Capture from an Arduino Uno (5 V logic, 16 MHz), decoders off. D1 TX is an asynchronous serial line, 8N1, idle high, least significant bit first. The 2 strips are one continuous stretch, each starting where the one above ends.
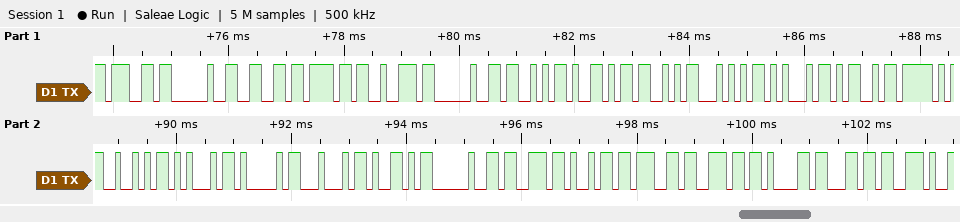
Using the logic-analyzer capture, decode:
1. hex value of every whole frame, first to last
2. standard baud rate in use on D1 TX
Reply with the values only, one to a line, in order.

67 20 66 6F 72 20 53 59 53 54 45 4D 5F 52 45 41 44 59 20 73 69 67 6E 61 6C 2E
9600 baud
